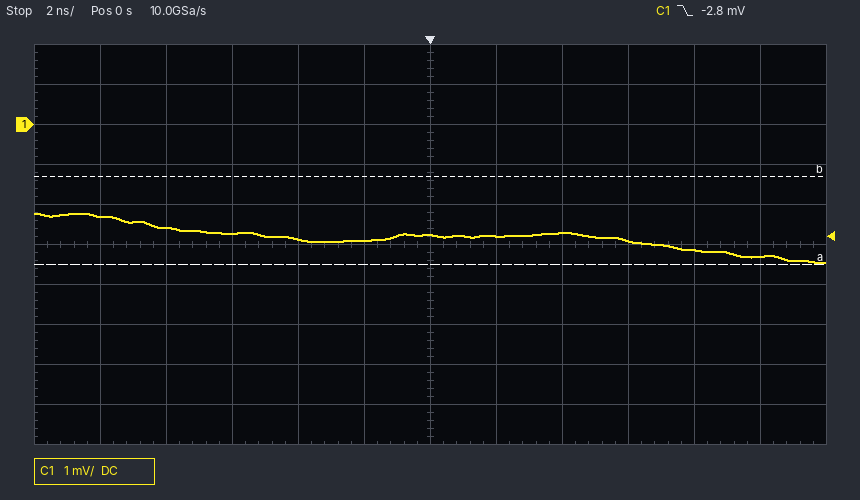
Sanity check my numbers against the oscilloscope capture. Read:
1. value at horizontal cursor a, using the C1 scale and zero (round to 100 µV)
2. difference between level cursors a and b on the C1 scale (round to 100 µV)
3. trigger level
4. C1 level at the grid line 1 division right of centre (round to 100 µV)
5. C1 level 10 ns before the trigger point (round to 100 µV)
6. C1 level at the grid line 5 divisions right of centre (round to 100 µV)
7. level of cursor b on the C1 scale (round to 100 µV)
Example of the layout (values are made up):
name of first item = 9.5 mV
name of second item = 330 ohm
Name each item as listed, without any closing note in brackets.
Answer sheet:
value at horizontal cursor a, using the C1 scale and zero = -3.5 mV
difference between level cursors a and b on the C1 scale = 2.2 mV
trigger level = -2.8 mV
C1 level at the grid line 1 division right of centre = -2.8 mV
C1 level 10 ns before the trigger point = -2.3 mV
C1 level at the grid line 5 divisions right of centre = -3.3 mV
level of cursor b on the C1 scale = -1.3 mV
